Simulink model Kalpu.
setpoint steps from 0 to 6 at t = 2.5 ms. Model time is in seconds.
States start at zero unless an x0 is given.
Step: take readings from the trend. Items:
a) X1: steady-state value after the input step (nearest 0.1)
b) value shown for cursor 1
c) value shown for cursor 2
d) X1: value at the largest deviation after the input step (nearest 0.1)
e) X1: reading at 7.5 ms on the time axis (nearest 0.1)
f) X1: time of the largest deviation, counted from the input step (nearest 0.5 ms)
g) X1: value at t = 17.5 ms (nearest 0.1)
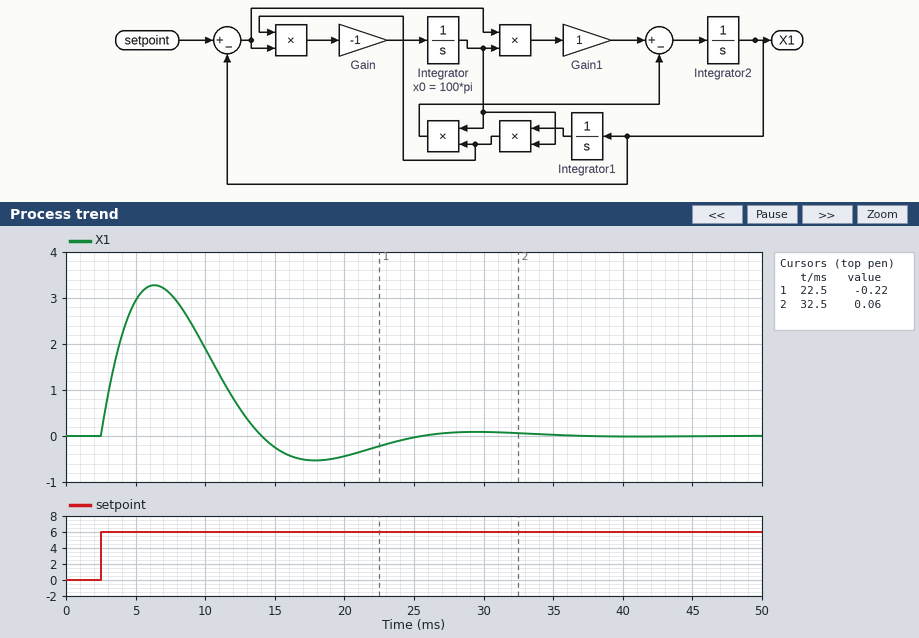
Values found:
0.0
-0.22
0.06
3.3
3.1
4.0 ms
-0.5
